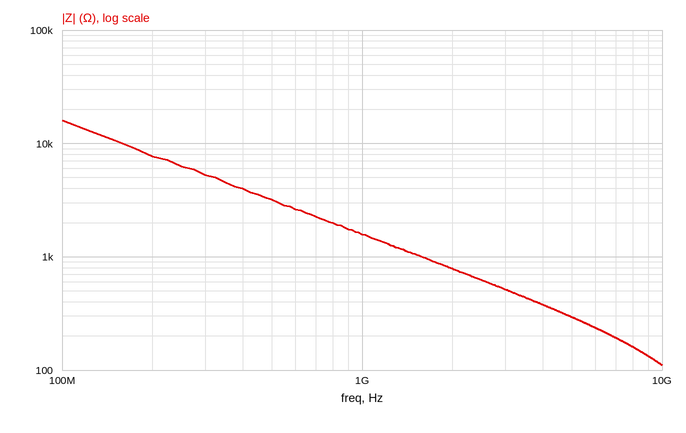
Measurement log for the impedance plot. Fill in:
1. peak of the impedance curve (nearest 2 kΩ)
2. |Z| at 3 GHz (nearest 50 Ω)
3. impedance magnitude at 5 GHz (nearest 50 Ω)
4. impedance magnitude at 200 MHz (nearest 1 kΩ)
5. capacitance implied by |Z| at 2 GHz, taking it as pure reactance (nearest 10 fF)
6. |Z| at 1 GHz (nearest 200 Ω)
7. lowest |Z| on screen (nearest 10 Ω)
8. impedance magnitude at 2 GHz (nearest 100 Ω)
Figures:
16 kΩ
500 Ω
300 Ω
8 kΩ
100 fF
1.6 kΩ
110 Ω
800 Ω
